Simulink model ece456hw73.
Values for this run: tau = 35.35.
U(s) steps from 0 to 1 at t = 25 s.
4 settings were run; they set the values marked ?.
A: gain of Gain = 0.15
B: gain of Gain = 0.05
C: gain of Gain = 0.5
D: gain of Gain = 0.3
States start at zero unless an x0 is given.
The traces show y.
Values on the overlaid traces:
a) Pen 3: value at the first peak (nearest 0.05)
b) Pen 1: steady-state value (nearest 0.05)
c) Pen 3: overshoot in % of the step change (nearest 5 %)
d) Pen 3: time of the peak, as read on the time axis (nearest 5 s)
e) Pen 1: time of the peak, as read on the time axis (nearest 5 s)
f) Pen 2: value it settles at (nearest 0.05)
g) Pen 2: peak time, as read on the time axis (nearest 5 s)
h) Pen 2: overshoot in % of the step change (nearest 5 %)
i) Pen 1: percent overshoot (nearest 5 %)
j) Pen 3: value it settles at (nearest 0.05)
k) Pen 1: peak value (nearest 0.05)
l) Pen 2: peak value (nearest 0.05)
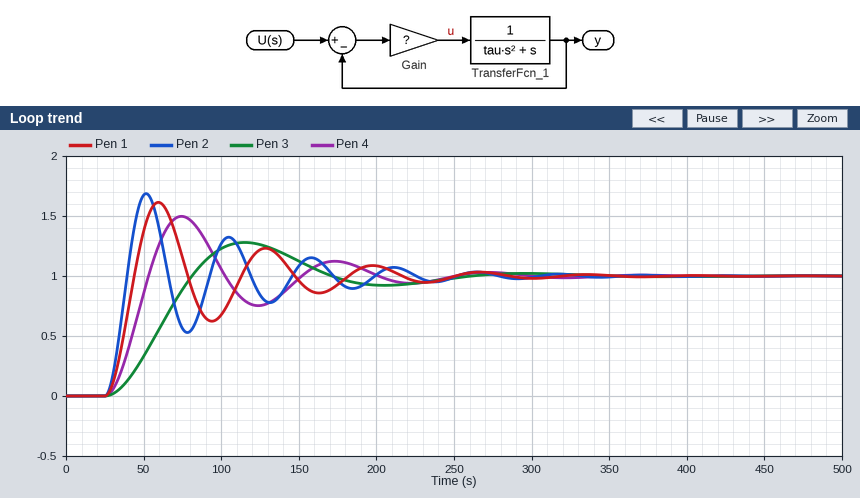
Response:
1.30
1.00
30 %
115 s
60 s
1.00
50 s
70 %
60 %
1.00
1.60
1.70
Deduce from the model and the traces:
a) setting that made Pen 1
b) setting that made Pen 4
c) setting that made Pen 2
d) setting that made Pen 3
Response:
D
A
C
B
